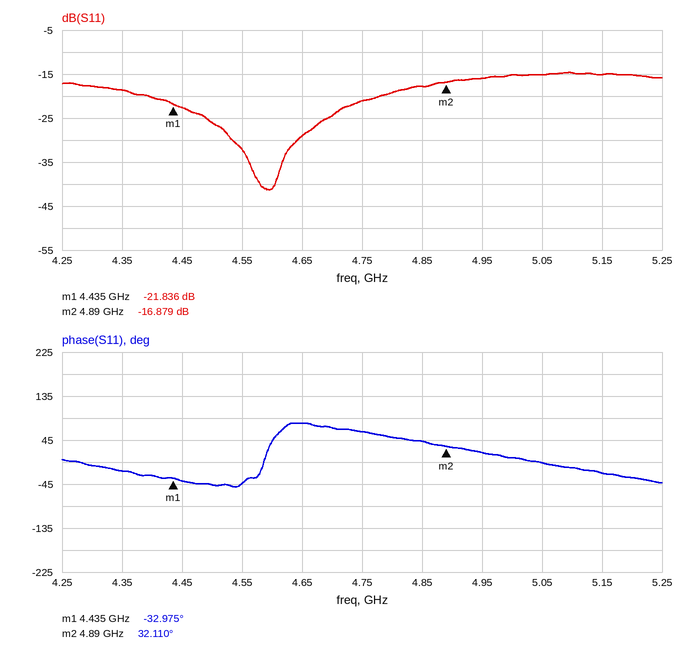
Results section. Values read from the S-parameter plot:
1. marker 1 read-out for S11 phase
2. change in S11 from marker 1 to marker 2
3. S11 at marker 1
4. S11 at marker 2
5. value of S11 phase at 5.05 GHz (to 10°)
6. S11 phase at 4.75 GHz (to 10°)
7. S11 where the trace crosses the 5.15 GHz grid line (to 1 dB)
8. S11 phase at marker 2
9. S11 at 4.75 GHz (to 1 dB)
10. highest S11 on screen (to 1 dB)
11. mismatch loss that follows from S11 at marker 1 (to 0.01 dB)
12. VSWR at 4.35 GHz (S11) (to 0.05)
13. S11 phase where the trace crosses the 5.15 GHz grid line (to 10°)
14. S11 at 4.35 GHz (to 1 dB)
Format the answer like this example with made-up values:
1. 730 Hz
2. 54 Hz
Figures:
1. -32.975°
2. 4.957 dB
3. -21.836 dB
4. -16.879 dB
5. 0°
6. 60°
7. -15 dB
8. 32.110°
9. -21 dB
10. -15 dB
11. 0.03 dB
12. 1.25
13. -20°
14. -19 dB
